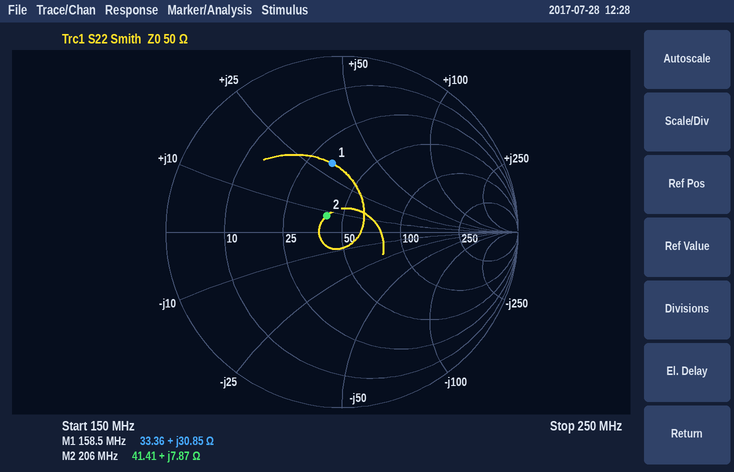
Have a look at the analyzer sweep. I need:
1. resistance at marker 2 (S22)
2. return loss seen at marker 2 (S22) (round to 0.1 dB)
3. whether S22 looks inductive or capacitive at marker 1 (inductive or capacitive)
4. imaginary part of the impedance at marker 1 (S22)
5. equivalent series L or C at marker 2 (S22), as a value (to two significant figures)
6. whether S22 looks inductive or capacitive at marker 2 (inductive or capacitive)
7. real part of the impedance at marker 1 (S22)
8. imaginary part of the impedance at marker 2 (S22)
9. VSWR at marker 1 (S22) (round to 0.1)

41.41 Ω
17.9 dB
inductive
+30.85 Ω
6.1 nH
inductive
33.36 Ω
+7.87 Ω
2.3
